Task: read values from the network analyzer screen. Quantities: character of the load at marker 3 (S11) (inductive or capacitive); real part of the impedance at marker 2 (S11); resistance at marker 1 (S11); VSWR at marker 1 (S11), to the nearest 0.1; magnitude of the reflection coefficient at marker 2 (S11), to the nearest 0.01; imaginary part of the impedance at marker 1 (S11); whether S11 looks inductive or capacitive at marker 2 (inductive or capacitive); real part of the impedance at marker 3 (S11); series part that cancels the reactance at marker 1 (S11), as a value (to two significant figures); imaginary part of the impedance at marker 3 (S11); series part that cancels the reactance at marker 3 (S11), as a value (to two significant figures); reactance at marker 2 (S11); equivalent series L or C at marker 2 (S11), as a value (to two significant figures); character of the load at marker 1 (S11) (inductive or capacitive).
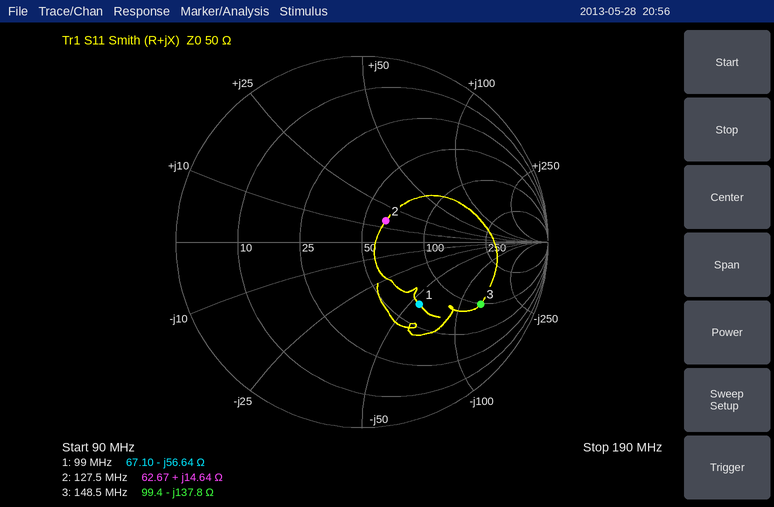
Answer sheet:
capacitive
62.67 Ω
67.10 Ω
2.7
0.17
-56.64 Ω
inductive
99.4 Ω
91 nH
-137.8 Ω
150 nH
+14.64 Ω
18 nH
capacitive
